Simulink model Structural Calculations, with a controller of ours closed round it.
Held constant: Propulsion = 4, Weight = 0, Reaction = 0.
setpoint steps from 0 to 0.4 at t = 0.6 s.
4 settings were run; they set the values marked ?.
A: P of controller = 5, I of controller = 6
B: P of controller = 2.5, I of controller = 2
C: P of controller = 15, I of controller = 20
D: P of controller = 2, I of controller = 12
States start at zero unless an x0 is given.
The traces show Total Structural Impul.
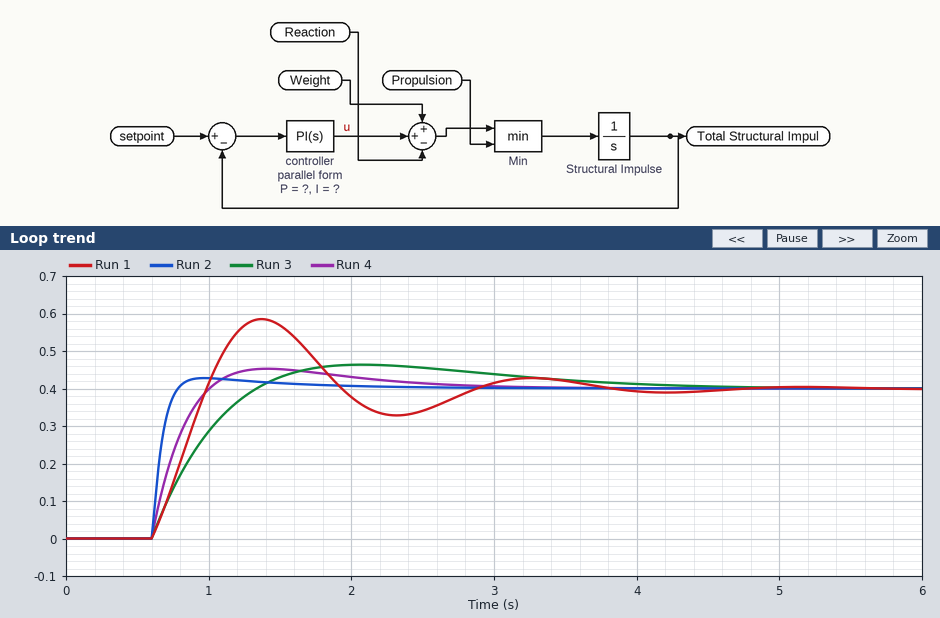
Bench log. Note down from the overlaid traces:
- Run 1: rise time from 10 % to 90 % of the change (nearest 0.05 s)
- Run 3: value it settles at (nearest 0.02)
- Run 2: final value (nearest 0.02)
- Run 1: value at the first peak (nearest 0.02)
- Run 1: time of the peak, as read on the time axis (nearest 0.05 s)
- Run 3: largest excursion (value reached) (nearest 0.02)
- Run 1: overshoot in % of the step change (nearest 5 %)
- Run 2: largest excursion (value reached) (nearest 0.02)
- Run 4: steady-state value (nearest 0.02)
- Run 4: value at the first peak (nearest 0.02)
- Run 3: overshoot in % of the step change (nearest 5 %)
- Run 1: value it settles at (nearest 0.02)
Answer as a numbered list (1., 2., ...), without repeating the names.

1. 0.30 s
2. 0.40
3. 0.40
4. 0.58
5. 1.35 s
6. 0.46
7. 45 %
8. 0.42
9. 0.40
10. 0.46
11. 15 %
12. 0.40
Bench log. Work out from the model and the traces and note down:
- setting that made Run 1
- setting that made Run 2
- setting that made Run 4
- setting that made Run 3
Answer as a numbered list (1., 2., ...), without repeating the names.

1. D
2. C
3. A
4. B
